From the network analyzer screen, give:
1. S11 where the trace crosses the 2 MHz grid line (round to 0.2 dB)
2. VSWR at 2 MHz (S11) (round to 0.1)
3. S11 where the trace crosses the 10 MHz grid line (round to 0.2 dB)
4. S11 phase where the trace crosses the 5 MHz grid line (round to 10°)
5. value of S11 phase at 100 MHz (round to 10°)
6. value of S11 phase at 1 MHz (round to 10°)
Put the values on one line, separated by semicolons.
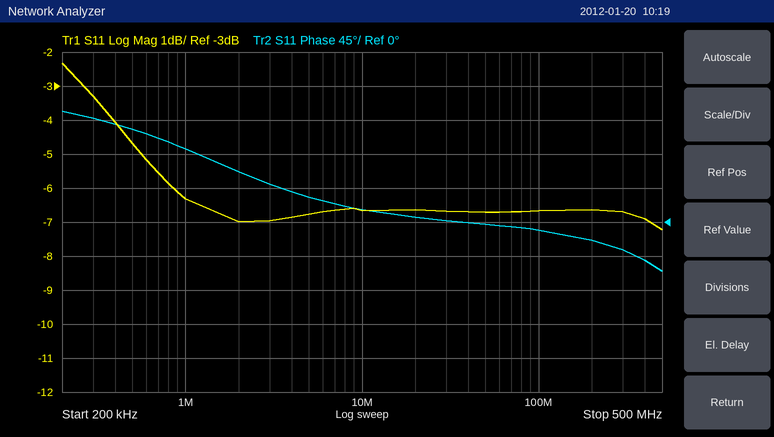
-7.0 dB; 2.6; -6.6 dB; 30°; -10°; 100°
